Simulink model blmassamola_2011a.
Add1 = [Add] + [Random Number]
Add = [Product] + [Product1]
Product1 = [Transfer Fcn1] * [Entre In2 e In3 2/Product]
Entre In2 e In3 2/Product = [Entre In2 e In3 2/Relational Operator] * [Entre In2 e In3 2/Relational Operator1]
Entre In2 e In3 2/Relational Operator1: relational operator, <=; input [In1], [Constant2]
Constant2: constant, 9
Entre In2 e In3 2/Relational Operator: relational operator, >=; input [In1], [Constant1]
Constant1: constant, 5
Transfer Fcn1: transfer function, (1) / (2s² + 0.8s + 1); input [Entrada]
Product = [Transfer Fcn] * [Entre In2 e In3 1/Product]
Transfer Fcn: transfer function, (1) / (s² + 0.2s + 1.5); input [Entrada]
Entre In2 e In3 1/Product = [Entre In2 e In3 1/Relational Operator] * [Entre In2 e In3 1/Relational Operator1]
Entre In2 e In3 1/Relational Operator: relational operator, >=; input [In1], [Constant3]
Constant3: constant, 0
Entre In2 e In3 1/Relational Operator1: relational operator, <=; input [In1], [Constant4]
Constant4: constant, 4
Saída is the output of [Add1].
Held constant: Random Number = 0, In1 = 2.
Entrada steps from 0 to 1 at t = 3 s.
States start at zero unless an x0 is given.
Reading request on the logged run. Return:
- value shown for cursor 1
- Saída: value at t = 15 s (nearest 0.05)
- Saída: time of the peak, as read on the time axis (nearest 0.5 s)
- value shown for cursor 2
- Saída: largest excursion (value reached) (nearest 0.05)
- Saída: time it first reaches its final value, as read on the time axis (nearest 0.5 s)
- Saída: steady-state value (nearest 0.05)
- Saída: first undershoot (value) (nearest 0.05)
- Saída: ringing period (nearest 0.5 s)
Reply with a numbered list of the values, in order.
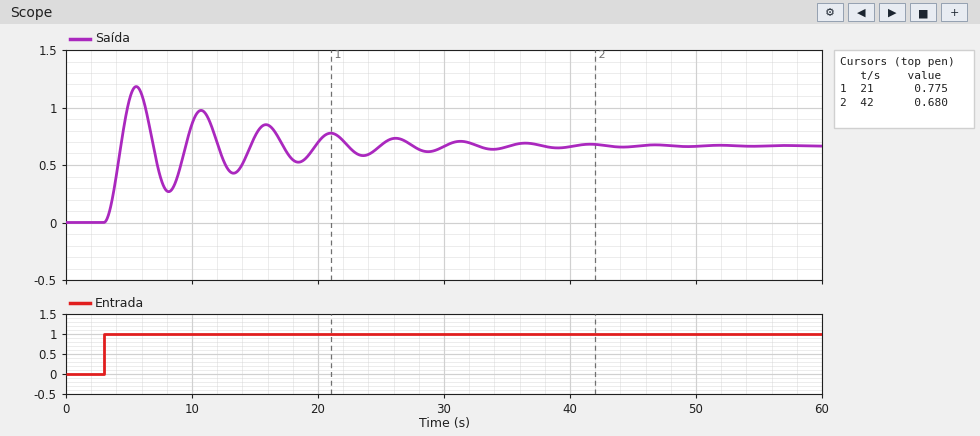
1. 0.775
2. 0.75
3. 5.5 s
4. 0.680
5. 1.20
6. 4.5 s
7. 0.65
8. 0.25
9. 5.0 s
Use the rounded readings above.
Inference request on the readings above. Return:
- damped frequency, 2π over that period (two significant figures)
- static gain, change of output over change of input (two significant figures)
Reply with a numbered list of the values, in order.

1. 1.3 rad/s
2. 0.65
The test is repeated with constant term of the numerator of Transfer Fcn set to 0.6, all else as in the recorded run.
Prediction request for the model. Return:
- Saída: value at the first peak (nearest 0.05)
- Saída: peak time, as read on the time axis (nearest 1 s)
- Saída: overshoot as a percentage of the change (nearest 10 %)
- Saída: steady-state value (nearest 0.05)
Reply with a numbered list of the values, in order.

1. 0.70
2. 6 s
3. 80 %
4. 0.40
